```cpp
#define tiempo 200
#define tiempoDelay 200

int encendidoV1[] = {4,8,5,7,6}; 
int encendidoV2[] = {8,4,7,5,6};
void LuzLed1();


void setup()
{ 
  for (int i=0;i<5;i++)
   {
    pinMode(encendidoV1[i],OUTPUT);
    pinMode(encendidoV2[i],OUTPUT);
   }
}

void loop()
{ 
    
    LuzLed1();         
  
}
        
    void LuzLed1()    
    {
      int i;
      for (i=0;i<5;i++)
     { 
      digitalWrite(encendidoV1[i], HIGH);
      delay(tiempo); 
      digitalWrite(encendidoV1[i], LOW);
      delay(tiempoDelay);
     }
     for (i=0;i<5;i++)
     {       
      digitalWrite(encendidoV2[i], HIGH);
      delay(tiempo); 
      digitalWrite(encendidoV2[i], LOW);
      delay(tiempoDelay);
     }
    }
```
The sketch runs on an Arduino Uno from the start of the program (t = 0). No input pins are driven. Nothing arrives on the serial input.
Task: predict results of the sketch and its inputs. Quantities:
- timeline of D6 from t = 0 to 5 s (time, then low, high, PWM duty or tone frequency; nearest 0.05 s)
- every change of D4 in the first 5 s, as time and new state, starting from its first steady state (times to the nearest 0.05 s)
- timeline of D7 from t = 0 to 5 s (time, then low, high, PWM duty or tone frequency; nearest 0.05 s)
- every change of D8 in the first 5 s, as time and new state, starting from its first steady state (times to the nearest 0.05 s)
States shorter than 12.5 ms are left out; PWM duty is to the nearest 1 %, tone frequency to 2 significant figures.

0 s low; 1.6 s high; 1.8 s low; 3.6 s high; 3.8 s low
0 s high; 0.2 s low; 2.4 s high; 2.6 s low; 4 s high; 4.2 s low
0 s low; 1.2 s high; 1.4 s low; 2.8 s high; 3 s low
0 s low; 0.4 s high; 0.6 s low; 2 s high; 2.2 s low; 4.4 s high; 4.6 s low
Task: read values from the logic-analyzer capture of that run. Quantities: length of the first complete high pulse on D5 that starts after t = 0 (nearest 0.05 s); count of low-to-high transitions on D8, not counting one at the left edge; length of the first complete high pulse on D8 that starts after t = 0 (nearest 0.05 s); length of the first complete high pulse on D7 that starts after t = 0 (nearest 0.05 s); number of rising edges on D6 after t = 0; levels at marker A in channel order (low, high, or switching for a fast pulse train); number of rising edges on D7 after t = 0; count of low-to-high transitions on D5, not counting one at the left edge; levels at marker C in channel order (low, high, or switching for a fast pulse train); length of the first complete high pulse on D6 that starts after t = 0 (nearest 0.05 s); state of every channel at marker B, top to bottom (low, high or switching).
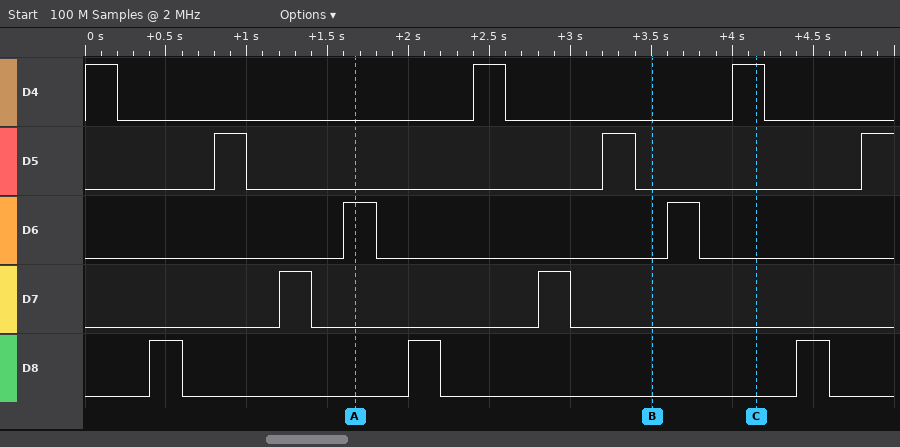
0.20 s
3
0.20 s
0.20 s
2
D4 low, D5 low, D6 high, D7 low, D8 low
2
3
D4 high, D5 low, D6 low, D7 low, D8 low
0.20 s
D4 low, D5 low, D6 low, D7 low, D8 low
